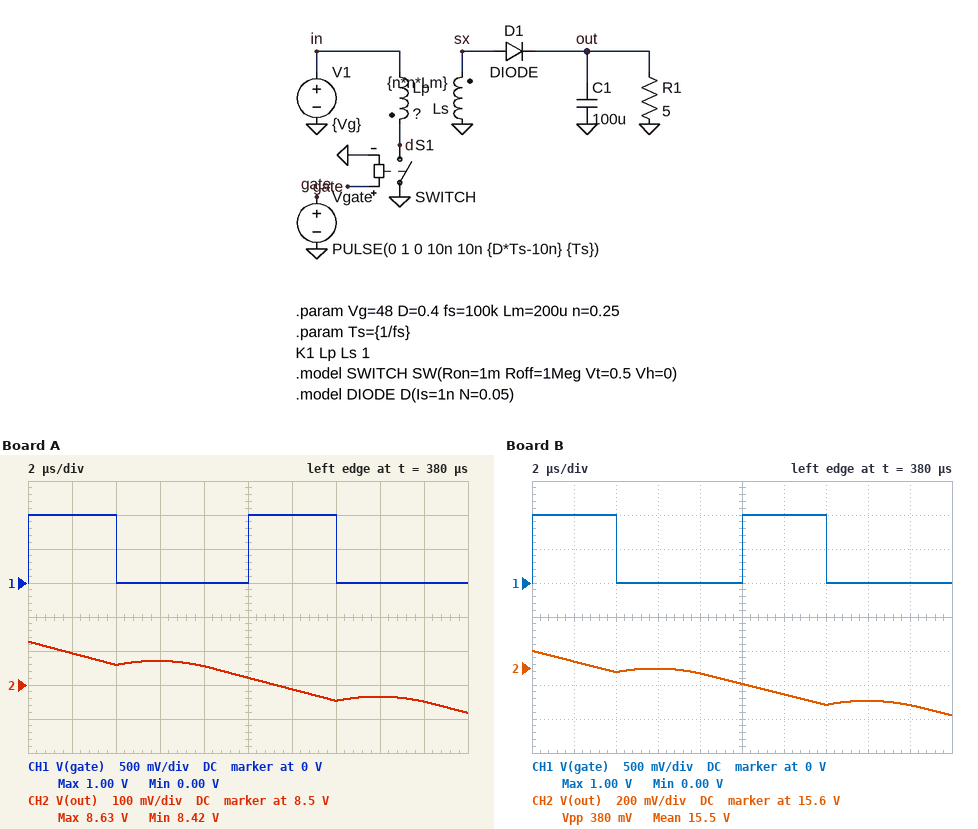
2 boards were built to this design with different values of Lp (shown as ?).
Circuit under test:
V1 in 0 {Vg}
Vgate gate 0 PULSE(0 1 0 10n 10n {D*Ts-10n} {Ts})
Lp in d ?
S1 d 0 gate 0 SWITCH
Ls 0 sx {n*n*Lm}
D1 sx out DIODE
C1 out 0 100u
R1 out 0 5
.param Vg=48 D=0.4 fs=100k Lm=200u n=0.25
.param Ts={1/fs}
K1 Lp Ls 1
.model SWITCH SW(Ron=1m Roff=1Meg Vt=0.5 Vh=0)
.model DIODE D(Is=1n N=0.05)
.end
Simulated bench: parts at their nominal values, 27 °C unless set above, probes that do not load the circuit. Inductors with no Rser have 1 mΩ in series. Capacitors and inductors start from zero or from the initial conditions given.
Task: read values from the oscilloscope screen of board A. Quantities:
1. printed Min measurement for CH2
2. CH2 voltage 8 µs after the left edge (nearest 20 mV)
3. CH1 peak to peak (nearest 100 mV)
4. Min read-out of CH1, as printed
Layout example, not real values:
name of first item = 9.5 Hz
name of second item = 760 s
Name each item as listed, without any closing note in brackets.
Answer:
printed Min measurement for CH2 = 8.42 V
CH2 voltage 8 µs after the left edge = 8.56 V
CH1 peak to peak = 1.0 V
Min read-out of CH1, as printed = 0.00 V
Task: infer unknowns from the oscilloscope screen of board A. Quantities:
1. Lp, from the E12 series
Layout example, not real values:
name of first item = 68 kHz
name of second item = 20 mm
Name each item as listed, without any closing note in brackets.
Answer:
Lp, from the E12 series = 330 µH
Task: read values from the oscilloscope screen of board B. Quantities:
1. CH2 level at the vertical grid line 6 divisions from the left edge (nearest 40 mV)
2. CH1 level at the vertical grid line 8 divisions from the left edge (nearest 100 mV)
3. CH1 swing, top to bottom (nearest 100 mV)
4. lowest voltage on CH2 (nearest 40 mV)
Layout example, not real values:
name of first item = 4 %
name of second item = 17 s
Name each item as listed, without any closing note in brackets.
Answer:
CH2 level at the vertical grid line 6 divisions from the left edge = 15.44 V
CH1 level at the vertical grid line 8 divisions from the left edge = 0 V
CH1 swing, top to bottom = 1.0 V
lowest voltage on CH2 = 15.32 V
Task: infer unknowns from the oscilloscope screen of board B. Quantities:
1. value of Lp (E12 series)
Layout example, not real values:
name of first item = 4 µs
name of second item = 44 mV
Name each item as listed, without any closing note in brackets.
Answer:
value of Lp = 100 µH
